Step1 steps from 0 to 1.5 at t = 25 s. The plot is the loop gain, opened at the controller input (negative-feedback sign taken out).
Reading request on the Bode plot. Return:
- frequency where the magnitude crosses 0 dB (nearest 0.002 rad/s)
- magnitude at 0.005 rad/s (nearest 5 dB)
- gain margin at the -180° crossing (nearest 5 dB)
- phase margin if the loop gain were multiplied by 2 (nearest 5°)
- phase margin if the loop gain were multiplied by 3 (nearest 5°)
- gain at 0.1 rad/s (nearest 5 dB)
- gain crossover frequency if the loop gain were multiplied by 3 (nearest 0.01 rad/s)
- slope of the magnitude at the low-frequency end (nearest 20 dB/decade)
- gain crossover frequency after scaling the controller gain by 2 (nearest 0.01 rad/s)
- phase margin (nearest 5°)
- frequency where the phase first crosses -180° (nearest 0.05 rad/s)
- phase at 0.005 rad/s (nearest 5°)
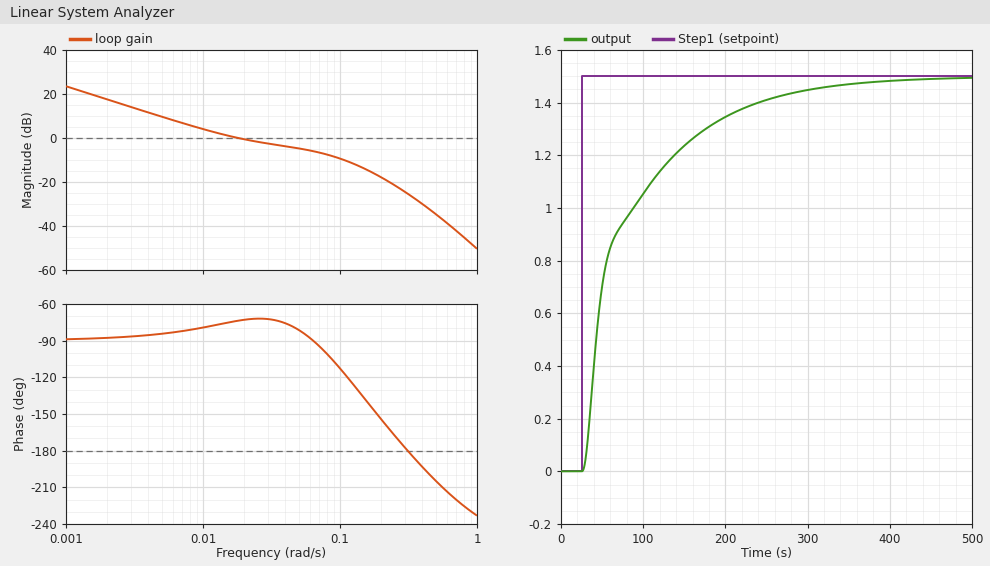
0.018 rad/s
10 dB
25 dB
90°
65°
-10 dB
0.10 rad/s
-20 dB/decade
0.06 rad/s
105°
0.30 rad/s
-85°
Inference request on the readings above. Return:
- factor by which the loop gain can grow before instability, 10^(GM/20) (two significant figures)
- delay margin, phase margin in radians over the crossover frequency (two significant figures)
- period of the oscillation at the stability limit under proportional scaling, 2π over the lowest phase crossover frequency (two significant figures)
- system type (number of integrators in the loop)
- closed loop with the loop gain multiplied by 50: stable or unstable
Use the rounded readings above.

18
100 s
21 s
1
unstable
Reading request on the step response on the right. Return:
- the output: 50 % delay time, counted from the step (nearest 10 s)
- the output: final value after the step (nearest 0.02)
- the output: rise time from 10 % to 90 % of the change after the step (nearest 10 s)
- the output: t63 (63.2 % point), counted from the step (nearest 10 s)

30 s
1.50
170 s
50 s
